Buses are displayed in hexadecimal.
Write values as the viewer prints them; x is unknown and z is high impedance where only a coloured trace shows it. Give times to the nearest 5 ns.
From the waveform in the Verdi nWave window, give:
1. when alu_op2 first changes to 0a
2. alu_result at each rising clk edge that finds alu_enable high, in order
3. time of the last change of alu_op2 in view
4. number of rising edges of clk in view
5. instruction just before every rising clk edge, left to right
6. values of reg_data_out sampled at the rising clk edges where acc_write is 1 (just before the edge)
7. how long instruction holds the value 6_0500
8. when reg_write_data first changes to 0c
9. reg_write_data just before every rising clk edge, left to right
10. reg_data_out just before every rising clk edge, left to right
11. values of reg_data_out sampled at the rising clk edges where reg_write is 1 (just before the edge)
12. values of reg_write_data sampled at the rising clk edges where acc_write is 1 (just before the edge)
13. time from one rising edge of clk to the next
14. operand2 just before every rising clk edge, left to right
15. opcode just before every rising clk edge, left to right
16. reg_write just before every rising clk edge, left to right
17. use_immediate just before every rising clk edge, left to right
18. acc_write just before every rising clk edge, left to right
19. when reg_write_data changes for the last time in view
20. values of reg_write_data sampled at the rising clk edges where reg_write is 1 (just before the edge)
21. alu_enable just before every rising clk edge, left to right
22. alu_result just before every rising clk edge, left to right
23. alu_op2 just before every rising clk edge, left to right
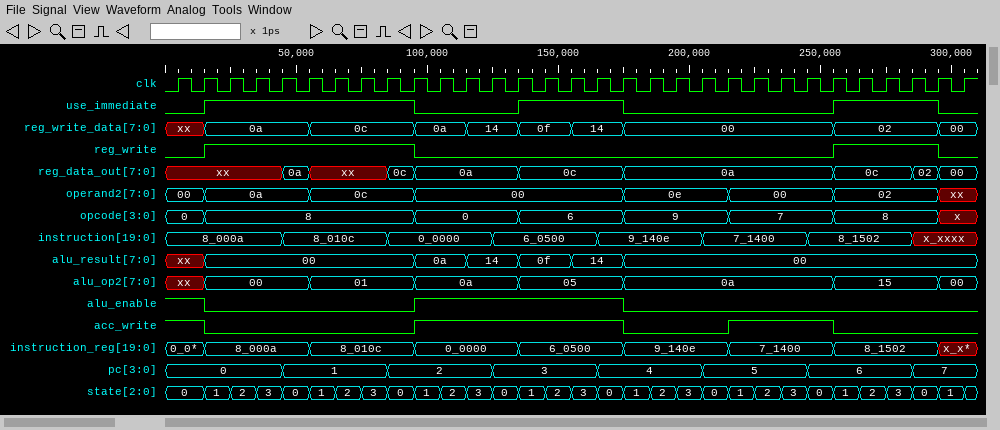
95 ns
xx, xx, 0a, 0a, 14, 14, 0f, 0f, 14, 14
295 ns
31
8_000a, 8_000a, 8_000a, 8_000a, 8_000a, 8_010c, 8_010c, 8_010c, 8_010c, 0_0000, 0_0000, 0_0000, 0_0000, 6_0500, 6_0500, 6_0500, 6_0500, 9_140e, 9_140e, 9_140e, 9_140e, 7_1400, 7_1400, 7_1400, 7_1400, 8_1502, 8_1502, 8_1502, 8_1502, x_xxxx, x_xxxx
xx, xx, 0a, 0a, 0a, 0a, 0c, 0c, 0c, 0c, 0a, 0a, 0a, 0a
40 ns
55 ns
xx, xx, 0a, 0a, 0a, 0a, 0c, 0c, 0c, 0c, 0a, 0a, 14, 14, 0f, 0f, 14, 14, 00, 00, 00, 00, 00, 00, 00, 00, 02, 02, 02, 02, 00
xx, xx, xx, xx, xx, 0a, xx, xx, xx, 0c, 0a, 0a, 0a, 0a, 0c, 0c, 0c, 0c, 0a, 0a, 0a, 0a, 0a, 0a, 0a, 0a, 0c, 0c, 0c, 02, 00
xx, xx, xx, 0a, xx, xx, xx, 0c, 0c, 0c, 0c, 02
xx, xx, 0a, 0a, 14, 14, 0f, 0f, 14, 14, 00, 00, 00, 00
10 ns
00, 00, 0a, 0a, 0a, 0a, 0c, 0c, 0c, 0c, 00, 00, 00, 00, 00, 00, 00, 00, 0e, 0e, 0e, 0e, 00, 00, 00, 00, 02, 02, 02, 02, xx
0, 0, 8, 8, 8, 8, 8, 8, 8, 8, 0, 0, 0, 0, 6, 6, 6, 6, 9, 9, 9, 9, 7, 7, 7, 7, 8, 8, 8, 8, x
0 0 1 1 1 1 1 1 1 1 0 0 0 0 0 0 0 0 0 0 0 0 0 0 0 0 1 1 1 1 0
0 0 1 1 1 1 1 1 1 1 0 0 0 0 1 1 1 1 0 0 0 0 0 0 0 0 1 1 1 1 0
1 1 0 0 0 0 0 0 0 0 1 1 1 1 1 1 1 1 0 0 0 0 1 1 1 1 0 0 0 0 0
295 ns
0a, 0a, 0a, 0a, 0c, 0c, 0c, 0c, 02, 02, 02, 02
1 1 0 0 0 0 0 0 0 0 1 1 1 1 1 1 1 1 0 0 0 0 0 0 0 0 0 0 0 0 0
xx, xx, 00, 00, 00, 00, 00, 00, 00, 00, 0a, 0a, 14, 14, 0f, 0f, 14, 14, 00, 00, 00, 00, 00, 00, 00, 00, 00, 00, 00, 00, 00
xx, xx, 00, 00, 00, 00, 01, 01, 01, 01, 0a, 0a, 0a, 0a, 05, 05, 05, 05, 0a, 0a, 0a, 0a, 0a, 0a, 0a, 0a, 15, 15, 15, 15, 00
